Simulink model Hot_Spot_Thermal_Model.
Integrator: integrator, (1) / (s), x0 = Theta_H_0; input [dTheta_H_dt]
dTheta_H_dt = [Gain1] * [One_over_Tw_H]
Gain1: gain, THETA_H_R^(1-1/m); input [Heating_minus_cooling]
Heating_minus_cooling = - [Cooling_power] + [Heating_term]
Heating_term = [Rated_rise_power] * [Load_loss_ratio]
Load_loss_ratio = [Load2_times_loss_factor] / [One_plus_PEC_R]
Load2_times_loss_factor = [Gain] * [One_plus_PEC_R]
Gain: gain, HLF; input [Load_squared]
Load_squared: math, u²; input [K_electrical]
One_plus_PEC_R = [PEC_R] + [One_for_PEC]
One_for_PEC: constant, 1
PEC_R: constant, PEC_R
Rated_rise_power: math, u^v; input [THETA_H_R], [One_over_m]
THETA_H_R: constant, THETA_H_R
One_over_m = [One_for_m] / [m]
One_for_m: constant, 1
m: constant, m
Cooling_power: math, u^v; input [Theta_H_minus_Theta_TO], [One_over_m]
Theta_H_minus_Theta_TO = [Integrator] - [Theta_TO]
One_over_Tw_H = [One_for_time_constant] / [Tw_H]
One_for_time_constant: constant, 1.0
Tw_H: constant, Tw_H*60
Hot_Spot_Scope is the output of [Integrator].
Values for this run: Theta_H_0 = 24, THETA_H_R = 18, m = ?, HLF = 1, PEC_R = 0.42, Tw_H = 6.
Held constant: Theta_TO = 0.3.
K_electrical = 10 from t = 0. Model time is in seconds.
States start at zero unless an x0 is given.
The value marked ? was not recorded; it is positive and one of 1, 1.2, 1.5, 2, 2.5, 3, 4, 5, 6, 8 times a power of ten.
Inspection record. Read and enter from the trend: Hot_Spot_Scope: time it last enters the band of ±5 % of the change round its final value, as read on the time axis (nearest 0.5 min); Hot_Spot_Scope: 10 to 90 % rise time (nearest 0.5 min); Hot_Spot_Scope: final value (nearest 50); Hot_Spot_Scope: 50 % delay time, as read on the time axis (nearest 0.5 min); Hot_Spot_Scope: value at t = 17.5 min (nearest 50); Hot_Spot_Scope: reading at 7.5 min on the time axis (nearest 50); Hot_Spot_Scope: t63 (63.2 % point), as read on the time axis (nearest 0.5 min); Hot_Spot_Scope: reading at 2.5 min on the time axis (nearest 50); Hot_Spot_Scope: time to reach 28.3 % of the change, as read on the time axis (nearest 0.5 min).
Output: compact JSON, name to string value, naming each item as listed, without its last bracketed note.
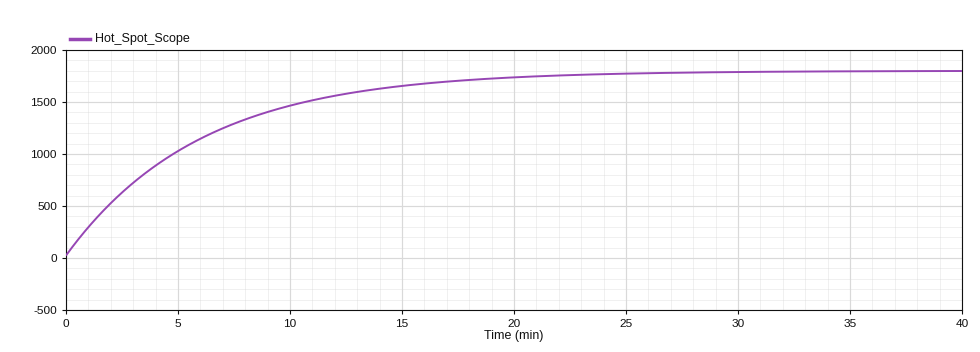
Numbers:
{"Hot_Spot_Scope: time it last enters the band of ±5 % of the change round its final value, as read on the time axis": "18.0 min", "Hot_Spot_Scope: 10 to 90 % rise time": "13.0 min", "Hot_Spot_Scope: final value": "1800", "Hot_Spot_Scope: 50 % delay time, as read on the time axis": "4.0 min", "Hot_Spot_Scope: value at t = 17.5 min": "1700", "Hot_Spot_Scope: reading at 7.5 min on the time axis": "1300", "Hot_Spot_Scope: t63 (63.2 % point), as read on the time axis": "6.0 min", "Hot_Spot_Scope: reading at 2.5 min on the time axis": "650", "Hot_Spot_Scope: time to reach 28.3 % of the change, as read on the time axis": "2.0 min"}
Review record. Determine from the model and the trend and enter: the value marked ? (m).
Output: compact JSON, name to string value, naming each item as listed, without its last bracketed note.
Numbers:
{"the value marked ?": "1"}
